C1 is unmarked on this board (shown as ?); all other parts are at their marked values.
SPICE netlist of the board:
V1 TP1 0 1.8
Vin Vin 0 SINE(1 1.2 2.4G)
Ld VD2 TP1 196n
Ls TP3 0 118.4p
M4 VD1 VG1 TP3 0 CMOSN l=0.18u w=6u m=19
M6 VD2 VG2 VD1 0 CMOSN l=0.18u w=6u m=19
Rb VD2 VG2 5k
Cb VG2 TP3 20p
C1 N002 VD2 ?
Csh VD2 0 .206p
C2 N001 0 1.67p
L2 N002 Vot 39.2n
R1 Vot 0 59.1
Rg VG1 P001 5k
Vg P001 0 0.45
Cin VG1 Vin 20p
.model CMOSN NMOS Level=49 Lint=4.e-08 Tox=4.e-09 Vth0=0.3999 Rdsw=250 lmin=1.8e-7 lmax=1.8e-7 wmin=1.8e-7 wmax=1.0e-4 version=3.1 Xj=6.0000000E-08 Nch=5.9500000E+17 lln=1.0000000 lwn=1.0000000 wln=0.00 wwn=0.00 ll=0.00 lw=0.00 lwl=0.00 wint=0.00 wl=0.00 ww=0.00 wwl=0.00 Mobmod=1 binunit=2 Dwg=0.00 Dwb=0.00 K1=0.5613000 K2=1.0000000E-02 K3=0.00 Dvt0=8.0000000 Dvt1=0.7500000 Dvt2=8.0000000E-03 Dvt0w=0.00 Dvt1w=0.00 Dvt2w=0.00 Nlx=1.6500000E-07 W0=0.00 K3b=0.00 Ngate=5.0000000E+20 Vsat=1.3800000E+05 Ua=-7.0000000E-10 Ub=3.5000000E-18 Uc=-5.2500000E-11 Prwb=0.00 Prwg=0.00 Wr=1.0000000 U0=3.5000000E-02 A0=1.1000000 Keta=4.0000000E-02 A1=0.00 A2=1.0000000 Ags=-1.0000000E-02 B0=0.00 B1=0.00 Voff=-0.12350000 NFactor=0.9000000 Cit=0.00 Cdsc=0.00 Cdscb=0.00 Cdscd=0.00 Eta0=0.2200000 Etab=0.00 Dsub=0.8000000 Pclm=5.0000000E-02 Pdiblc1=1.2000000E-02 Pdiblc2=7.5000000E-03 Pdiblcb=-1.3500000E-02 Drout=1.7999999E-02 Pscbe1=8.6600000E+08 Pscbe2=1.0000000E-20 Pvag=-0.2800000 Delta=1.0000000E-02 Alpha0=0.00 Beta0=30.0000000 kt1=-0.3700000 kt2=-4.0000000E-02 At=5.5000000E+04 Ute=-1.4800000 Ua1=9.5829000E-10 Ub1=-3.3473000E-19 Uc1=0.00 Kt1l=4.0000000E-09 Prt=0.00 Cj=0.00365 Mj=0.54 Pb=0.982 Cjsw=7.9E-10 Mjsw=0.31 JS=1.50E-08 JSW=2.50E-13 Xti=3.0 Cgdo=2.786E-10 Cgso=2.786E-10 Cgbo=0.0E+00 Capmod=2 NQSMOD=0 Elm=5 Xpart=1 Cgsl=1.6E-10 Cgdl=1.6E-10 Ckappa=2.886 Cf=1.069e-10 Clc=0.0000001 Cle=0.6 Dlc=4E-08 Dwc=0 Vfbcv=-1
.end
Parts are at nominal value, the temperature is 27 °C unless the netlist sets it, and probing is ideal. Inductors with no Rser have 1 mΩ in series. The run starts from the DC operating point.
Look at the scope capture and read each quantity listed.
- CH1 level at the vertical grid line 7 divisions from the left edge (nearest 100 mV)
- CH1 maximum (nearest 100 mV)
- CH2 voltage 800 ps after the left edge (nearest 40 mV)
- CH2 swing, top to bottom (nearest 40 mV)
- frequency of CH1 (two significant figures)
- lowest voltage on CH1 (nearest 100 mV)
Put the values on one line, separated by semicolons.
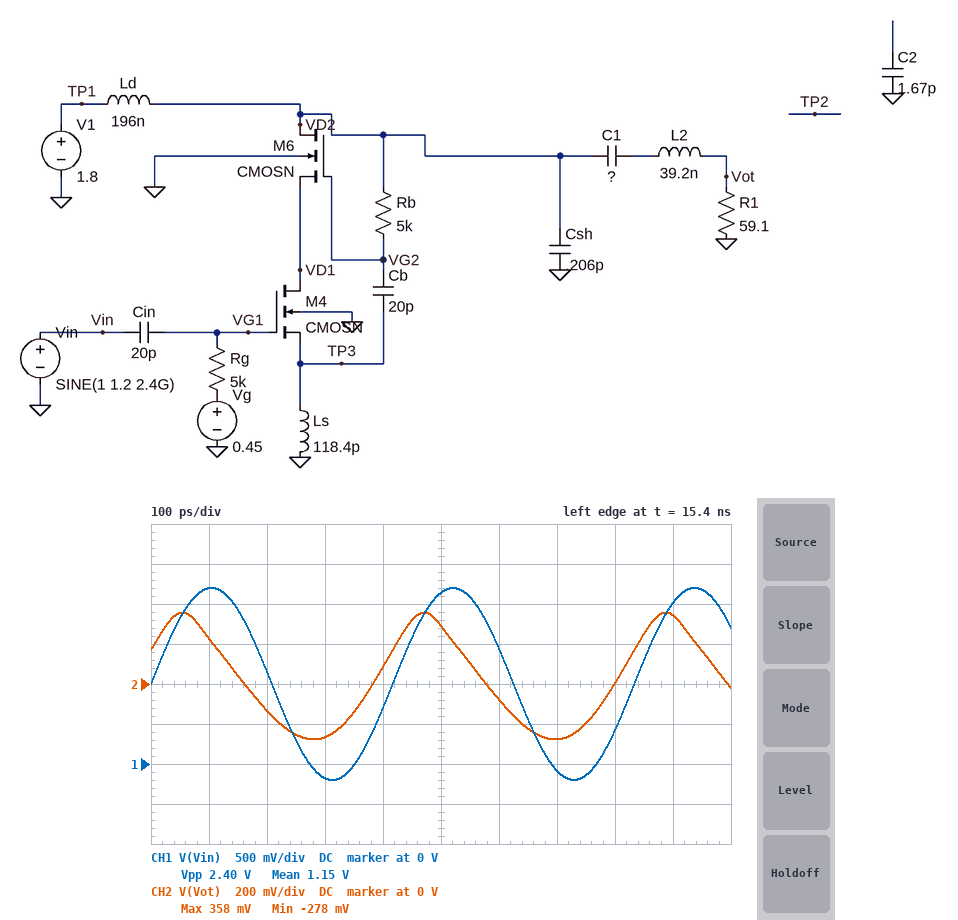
-100 mV; 2.2 V; 0 V; 640 mV; 2.4 GHz; -200 mV
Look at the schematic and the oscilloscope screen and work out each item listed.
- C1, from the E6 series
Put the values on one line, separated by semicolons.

470 fF
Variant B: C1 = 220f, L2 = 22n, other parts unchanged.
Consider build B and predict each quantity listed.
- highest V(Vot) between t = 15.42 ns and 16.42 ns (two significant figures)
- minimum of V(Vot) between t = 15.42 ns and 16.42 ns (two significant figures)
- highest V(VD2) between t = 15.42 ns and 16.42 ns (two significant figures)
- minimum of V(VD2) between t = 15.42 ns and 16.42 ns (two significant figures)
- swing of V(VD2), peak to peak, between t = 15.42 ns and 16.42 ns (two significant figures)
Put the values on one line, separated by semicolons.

1.3 V; -1.2 V; 3.7 V; 360 mV; 3.3 V
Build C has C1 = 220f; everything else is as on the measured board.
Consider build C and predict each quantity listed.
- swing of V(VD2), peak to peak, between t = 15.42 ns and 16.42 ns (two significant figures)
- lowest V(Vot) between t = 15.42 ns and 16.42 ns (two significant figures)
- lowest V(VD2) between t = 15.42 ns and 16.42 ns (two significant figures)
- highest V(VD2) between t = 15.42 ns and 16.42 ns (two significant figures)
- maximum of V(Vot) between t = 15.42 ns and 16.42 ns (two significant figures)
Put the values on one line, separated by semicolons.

4.6 V; -440 mV; -240 mV; 4.3 V; 510 mV
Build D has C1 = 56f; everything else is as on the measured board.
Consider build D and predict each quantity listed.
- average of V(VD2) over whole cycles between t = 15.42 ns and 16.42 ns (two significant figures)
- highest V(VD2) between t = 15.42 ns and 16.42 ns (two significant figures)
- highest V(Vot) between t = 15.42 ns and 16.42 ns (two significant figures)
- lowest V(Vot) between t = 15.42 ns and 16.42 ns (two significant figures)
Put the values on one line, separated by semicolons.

1.8 V; 5.1 V; 270 mV; -240 mV
